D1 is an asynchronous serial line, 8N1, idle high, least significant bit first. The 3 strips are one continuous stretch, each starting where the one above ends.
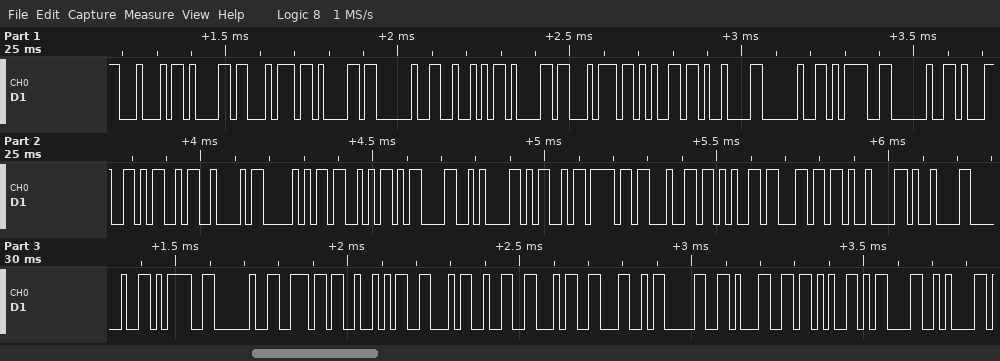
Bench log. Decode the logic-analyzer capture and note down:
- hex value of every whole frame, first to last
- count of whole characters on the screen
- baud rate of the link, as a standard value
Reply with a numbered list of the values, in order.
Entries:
1. 44 61 74 61 20 52 61 74 65 09 20 3D 20 31 4D 42 50 53 0D 0A 4D 6F 64 65 6C 09 09 20 3D 20 6E 52 46 32 34 4C 30 31 2B 0D 0A
2. 41
3. 57600 baud
